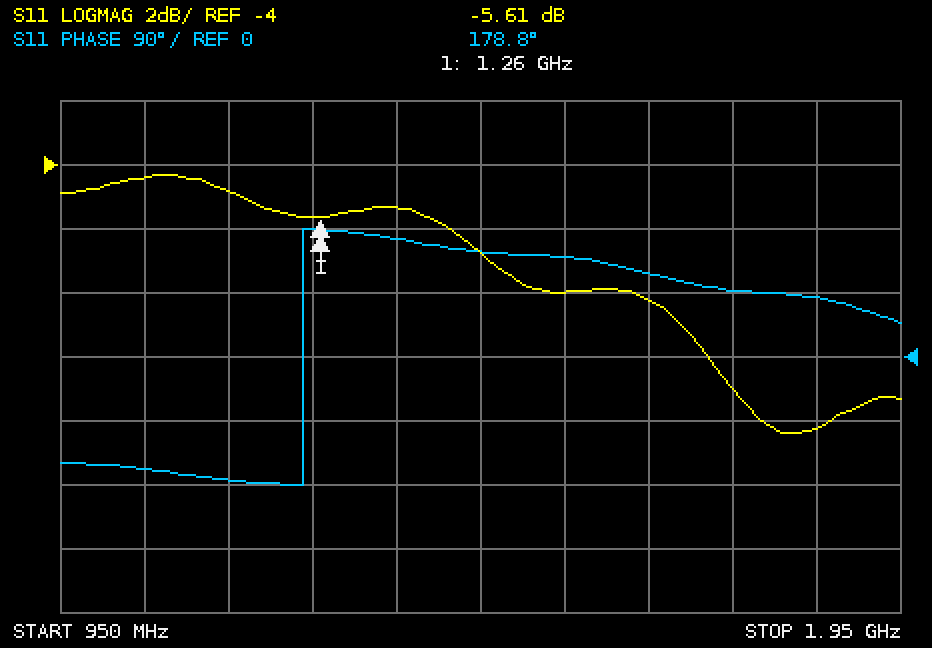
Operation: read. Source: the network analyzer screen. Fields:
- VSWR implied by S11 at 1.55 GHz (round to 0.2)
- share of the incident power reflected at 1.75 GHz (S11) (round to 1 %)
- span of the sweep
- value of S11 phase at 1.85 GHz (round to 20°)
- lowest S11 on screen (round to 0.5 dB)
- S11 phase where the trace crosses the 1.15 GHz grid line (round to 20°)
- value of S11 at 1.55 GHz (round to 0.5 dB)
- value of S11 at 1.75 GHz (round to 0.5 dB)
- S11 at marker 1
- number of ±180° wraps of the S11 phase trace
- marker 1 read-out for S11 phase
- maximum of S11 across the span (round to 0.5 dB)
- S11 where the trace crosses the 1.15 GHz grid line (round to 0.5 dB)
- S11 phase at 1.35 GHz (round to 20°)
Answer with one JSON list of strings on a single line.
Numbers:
["2.4", "8 %", "1 GHz", "80°", "-12.5 dB", "-180°", "-8.0 dB", "-11.0 dB", "-5.61 dB", "1", "178.8°", "-4.5 dB", "-5.0 dB", "160°"]
